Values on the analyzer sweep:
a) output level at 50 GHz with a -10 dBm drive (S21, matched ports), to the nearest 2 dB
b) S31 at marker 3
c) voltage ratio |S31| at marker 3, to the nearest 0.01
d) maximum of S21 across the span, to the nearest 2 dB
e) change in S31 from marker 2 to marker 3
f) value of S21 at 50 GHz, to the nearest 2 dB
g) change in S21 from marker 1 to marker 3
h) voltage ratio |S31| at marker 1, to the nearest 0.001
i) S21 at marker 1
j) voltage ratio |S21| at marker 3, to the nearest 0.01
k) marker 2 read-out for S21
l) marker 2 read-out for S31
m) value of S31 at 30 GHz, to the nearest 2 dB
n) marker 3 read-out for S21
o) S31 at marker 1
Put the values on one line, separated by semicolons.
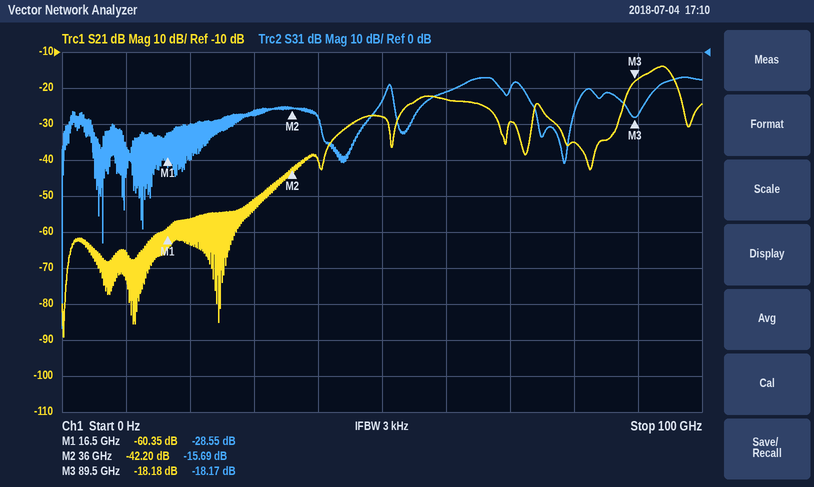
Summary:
-38 dBm; -18.17 dB; 0.12; -14 dB; -2.48 dB; -28 dB; 42.17 dB; 0.037; -60.35 dB; 0.12; -42.20 dB; -15.69 dB; -16 dB; -18.18 dB; -28.55 dB
